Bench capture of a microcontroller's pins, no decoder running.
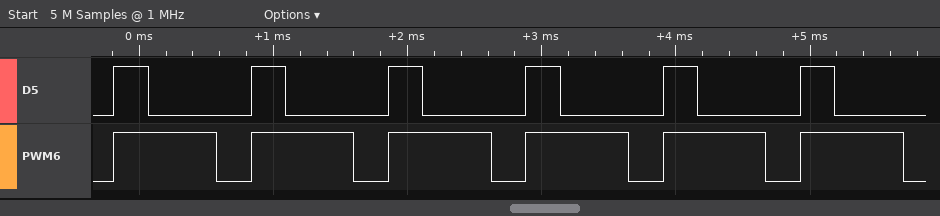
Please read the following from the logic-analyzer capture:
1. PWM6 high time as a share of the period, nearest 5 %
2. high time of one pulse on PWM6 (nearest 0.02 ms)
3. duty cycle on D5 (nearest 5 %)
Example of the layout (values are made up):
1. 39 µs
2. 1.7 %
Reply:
1. 75 %
2. 0.76 ms
3. 25 %
